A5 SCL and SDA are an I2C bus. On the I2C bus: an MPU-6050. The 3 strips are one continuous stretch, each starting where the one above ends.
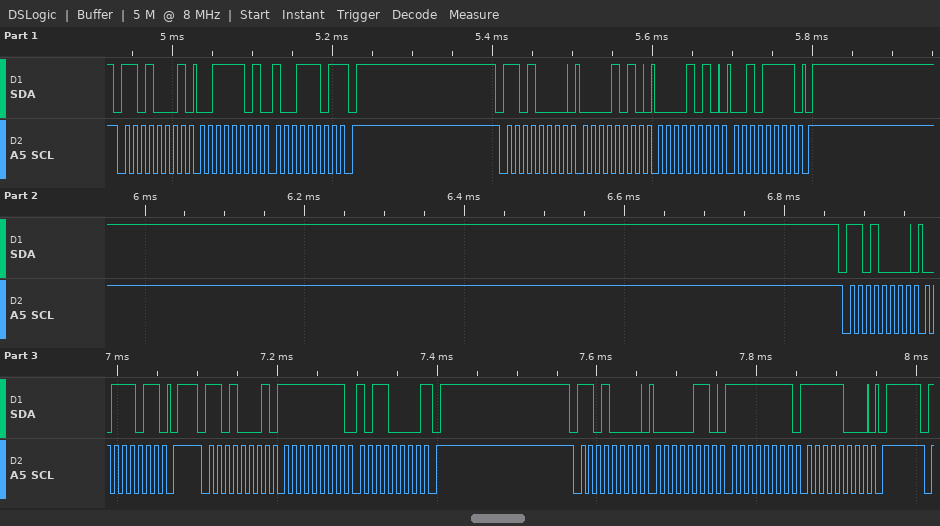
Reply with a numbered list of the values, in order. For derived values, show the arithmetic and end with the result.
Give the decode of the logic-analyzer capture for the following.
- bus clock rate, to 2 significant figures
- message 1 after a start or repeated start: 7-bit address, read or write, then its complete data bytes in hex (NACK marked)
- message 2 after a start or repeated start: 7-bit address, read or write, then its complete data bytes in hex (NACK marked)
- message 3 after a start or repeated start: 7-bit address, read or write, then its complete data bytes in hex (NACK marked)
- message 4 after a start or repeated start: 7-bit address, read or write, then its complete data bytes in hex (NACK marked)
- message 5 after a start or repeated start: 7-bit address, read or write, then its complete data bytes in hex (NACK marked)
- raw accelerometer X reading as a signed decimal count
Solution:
1. 100 kHz
2. 0x68 read: 3D 9D NACK
3. 0x68 write: 0A 0A 2F
4. 0x68 write: 3B
5. 0x68 read: FF B0 NACK
6. 0x68 write: 06 FF F8
7. 0xFFB0 = -80
